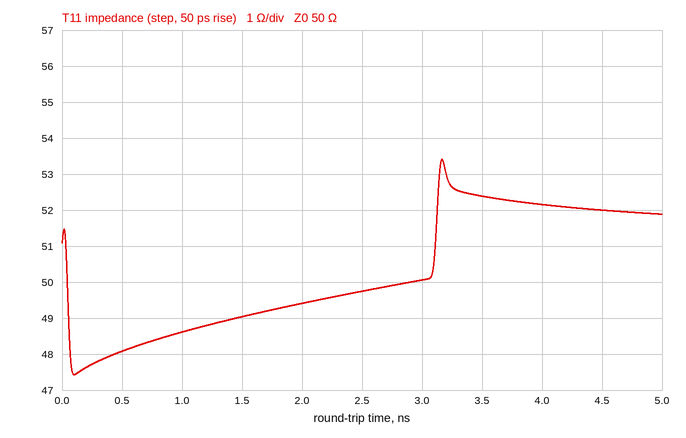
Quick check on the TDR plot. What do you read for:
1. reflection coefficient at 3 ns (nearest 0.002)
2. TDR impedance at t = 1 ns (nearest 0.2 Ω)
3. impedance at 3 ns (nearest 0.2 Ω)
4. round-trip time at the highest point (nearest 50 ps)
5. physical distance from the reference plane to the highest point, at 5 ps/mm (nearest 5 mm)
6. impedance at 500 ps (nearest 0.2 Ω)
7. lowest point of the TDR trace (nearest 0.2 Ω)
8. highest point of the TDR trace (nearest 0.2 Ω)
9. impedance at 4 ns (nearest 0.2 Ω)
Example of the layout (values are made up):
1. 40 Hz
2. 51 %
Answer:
1. 0.000
2. 48.6 Ω
3. 50.0 Ω
4. 3.15 ns
5. 315 mm
6. 48.0 Ω
7. 47.4 Ω
8. 53.4 Ω
9. 52.2 Ω
